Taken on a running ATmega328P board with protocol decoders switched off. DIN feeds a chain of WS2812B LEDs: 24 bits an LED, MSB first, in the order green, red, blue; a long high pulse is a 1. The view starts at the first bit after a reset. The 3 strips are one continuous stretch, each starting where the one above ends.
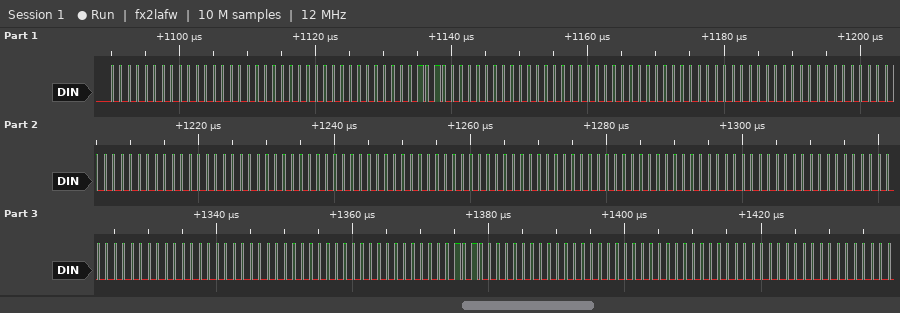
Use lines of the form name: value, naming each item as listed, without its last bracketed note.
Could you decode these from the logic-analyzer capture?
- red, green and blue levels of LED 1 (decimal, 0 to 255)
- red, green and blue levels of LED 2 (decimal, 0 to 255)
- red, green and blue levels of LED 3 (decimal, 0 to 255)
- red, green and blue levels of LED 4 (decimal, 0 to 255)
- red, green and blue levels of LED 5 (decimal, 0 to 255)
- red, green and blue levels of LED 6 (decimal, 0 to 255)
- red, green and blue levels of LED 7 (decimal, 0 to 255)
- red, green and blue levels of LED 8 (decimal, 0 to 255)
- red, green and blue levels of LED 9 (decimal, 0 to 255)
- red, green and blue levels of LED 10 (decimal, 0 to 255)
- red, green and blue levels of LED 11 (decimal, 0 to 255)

red, green and blue levels of LED 1: 0, 0, 0
red, green and blue levels of LED 2: 10, 0, 0
red, green and blue levels of LED 3: 0, 0, 0
red, green and blue levels of LED 4: 0, 0, 0
red, green and blue levels of LED 5: 0, 0, 0
red, green and blue levels of LED 6: 0, 0, 0
red, green and blue levels of LED 7: 0, 0, 0
red, green and blue levels of LED 8: 0, 0, 0
red, green and blue levels of LED 9: 0, 0, 0
red, green and blue levels of LED 10: 10, 0, 0
red, green and blue levels of LED 11: 0, 0, 0
